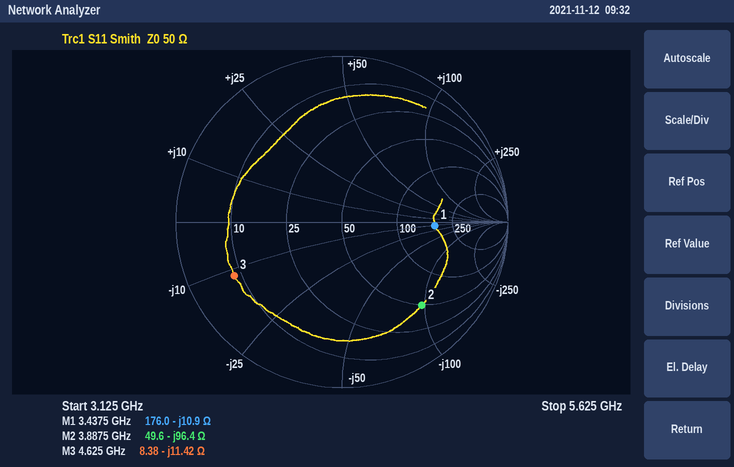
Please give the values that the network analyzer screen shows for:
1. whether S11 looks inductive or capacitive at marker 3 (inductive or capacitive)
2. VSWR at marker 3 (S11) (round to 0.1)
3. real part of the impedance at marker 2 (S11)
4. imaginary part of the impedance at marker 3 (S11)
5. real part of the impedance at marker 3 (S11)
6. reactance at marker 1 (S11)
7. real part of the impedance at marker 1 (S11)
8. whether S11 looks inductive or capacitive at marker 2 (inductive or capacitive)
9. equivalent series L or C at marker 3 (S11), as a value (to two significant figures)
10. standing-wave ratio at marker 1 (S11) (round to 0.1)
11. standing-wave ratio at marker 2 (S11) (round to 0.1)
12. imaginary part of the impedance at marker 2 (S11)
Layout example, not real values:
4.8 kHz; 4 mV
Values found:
capacitive; 6.3; 49.6 Ω; -11.42 Ω; 8.38 Ω; -10.9 Ω; 176.0 Ω; capacitive; 3.0 pF; 3.5; 5.6; -96.4 Ω
